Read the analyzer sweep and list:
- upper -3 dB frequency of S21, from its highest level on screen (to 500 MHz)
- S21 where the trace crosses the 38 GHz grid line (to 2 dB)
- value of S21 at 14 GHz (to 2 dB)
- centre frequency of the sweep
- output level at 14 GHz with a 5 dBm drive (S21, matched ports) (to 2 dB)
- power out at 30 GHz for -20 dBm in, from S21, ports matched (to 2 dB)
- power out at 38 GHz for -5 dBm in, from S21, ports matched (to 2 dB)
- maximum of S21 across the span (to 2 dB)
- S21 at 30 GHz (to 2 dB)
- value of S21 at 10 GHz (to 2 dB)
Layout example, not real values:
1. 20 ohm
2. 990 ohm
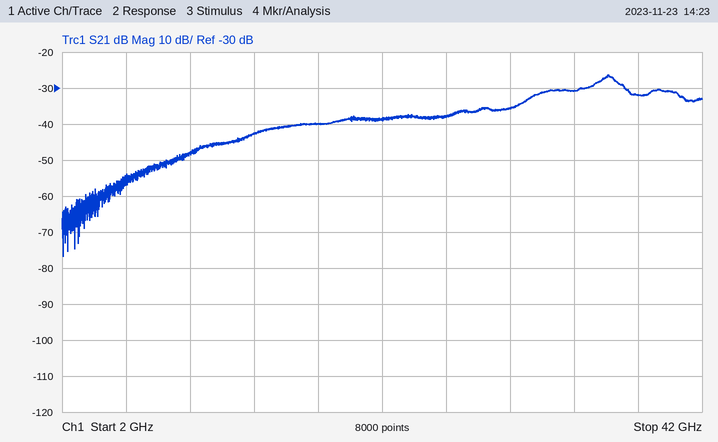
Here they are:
1. 37.0 GHz
2. -32 dB
3. -42 dB
4. 22 GHz
5. -38 dBm
6. -56 dBm
7. -36 dBm
8. -26 dB
9. -36 dB
10. -48 dB
